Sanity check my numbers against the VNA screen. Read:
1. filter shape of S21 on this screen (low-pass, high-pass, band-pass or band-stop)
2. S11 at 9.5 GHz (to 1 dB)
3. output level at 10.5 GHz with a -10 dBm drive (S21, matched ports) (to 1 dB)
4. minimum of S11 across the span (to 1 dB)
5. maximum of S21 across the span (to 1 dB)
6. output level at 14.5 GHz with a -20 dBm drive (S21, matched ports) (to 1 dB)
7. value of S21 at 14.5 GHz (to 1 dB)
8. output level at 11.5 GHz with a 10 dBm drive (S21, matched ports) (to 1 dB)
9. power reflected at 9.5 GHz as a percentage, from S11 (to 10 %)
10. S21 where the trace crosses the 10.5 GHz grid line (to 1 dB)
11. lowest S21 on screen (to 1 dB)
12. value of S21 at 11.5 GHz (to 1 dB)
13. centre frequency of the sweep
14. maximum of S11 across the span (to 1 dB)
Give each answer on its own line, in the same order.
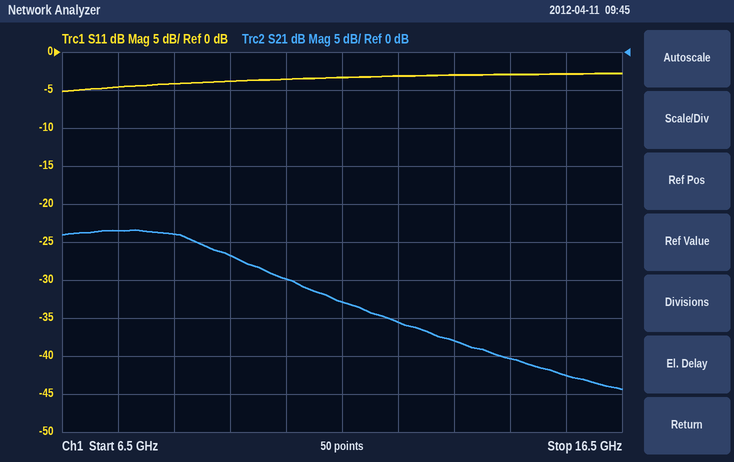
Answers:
low-pass
-4 dB
-40 dBm
-5 dB
-23 dB
-60 dBm
-40 dB
-23 dBm
40 %
-30 dB
-44 dB
-33 dB
11.5 GHz
-3 dB
